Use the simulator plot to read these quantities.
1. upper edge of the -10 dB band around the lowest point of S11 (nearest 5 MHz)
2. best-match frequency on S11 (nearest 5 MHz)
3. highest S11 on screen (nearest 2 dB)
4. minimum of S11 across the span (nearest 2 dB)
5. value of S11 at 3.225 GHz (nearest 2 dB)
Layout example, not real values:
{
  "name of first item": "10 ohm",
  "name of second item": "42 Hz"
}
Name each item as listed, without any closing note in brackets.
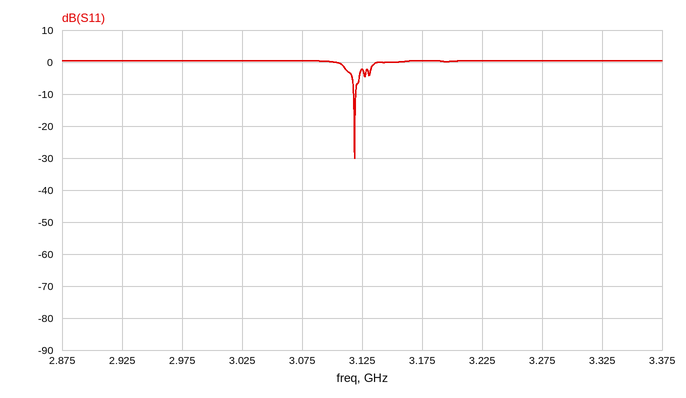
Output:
{
  "upper edge of the -10 dB band around the lowest point of S11": "3.120 GHz",
  "best-match frequency on S11": "3.120 GHz",
  "highest S11 on screen": "0 dB",
  "minimum of S11 across the span": "-30 dB",
  "value of S11 at 3.225 GHz": "0 dB"
}
